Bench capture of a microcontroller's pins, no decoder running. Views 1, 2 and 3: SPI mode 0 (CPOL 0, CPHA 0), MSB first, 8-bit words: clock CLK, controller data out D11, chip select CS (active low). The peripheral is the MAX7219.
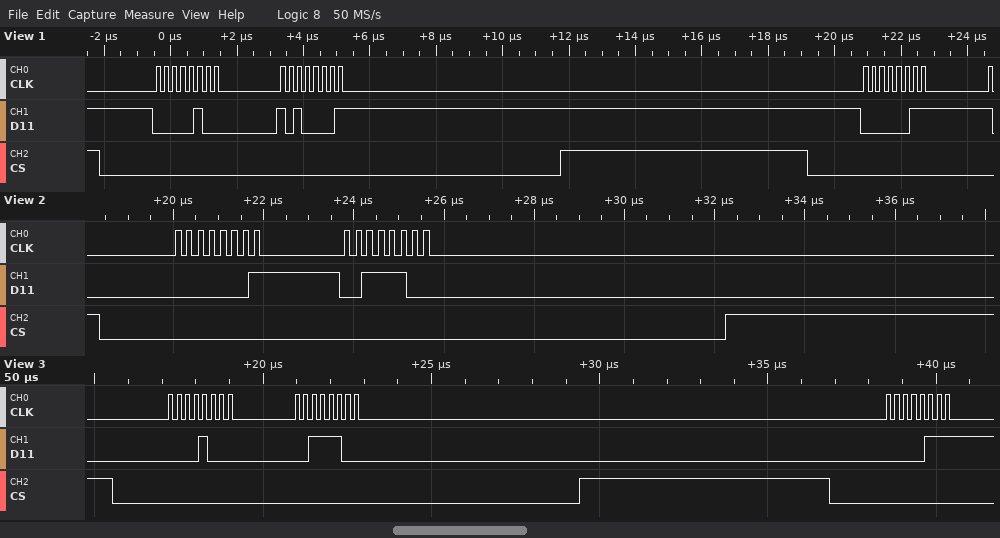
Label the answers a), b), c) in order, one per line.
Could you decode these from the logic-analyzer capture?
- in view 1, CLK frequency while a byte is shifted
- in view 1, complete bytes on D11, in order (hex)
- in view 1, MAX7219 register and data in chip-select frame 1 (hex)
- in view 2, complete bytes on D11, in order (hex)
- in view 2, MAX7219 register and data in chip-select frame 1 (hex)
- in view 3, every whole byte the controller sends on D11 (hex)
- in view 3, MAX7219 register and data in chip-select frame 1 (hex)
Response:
a) 4 MHz
b) 04 A1 03
c) register 0x4, data 0xA1
d) 01 3C
e) register 0x1, data 0x3C
f) 08 3C 07
g) register 0x8, data 0x3C
